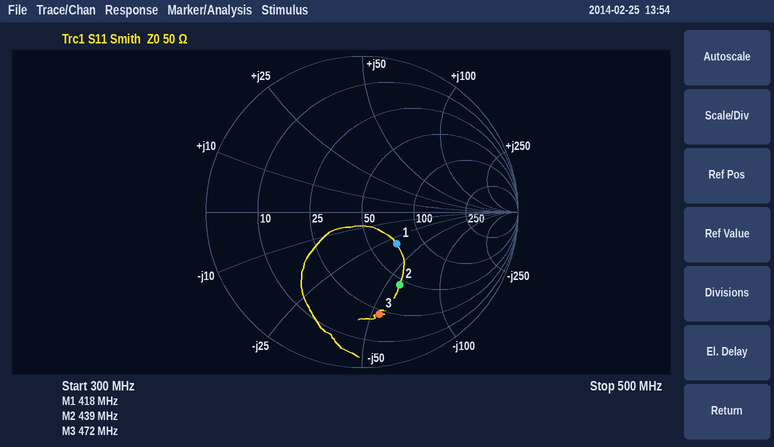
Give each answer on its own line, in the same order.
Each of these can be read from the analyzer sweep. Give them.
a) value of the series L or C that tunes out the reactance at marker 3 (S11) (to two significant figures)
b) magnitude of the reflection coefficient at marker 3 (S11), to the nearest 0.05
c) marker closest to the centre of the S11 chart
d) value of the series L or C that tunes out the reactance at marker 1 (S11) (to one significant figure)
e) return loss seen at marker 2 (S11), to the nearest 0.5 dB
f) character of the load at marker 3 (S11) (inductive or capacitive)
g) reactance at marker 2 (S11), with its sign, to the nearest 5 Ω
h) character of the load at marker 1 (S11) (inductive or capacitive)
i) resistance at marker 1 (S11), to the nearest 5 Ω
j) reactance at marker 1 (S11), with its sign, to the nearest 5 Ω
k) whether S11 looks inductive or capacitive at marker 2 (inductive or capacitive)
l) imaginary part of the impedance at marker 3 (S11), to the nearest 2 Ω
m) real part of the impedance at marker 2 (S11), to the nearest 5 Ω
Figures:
18 nH
0.65
marker 1
10 nH
5.5 dB
capacitive
-60 Ω
capacitive
70 Ω
-30 Ω
capacitive
-54 Ω
45 Ω
